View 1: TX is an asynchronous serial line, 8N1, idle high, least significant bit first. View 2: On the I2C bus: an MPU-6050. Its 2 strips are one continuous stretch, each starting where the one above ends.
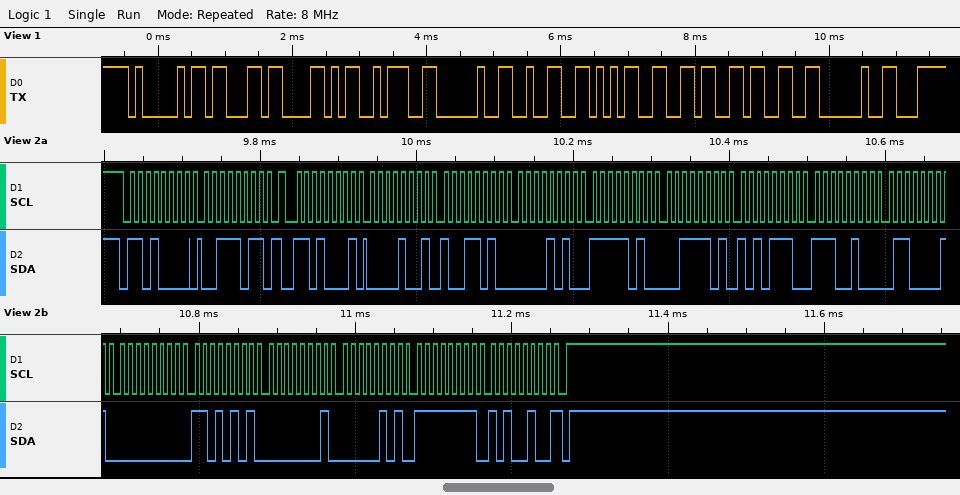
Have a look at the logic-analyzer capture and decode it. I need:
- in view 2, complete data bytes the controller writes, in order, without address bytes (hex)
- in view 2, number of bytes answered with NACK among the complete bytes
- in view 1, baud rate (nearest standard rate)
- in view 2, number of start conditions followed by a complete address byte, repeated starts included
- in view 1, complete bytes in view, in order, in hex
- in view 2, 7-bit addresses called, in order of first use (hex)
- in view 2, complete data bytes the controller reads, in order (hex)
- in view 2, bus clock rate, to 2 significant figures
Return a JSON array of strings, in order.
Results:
["3B", "1", "9600 baud", "2", "41 63 58 3A 20 32 35 36 33 20", "0x68", "09 9A 0A FA 3D AE E4 61 00 D5 01 05 FF A4", "100 kHz"]
